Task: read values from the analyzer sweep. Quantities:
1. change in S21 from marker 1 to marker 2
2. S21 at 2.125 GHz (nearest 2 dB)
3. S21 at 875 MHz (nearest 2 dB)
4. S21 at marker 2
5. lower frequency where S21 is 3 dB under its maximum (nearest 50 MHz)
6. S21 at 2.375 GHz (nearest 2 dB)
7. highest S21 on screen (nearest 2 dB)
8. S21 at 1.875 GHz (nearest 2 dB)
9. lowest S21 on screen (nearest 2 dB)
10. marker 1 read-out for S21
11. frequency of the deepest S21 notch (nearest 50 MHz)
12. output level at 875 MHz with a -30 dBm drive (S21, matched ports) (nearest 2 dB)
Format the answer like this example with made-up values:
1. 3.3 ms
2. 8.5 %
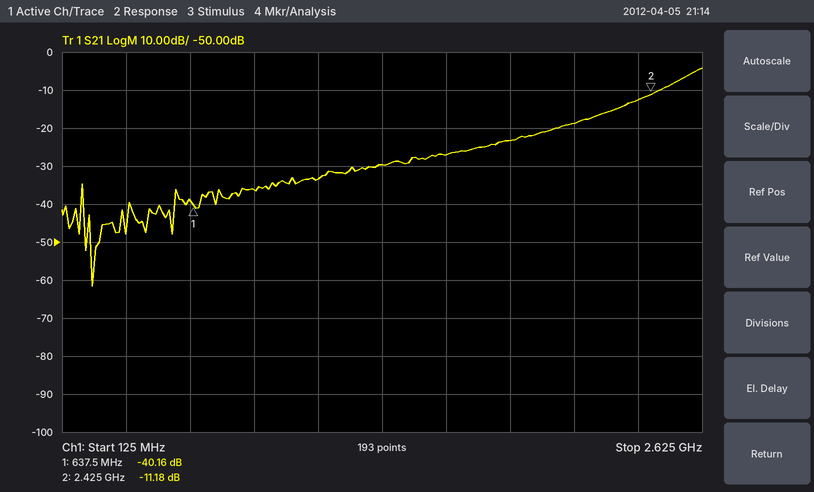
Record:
1. 28.98 dB
2. -18 dB
3. -36 dB
4. -11.18 dB
5. 2.55 GHz
6. -12 dB
7. -4 dB
8. -24 dB
9. -62 dB
10. -40.16 dB
11. 250 MHz
12. -66 dBm
